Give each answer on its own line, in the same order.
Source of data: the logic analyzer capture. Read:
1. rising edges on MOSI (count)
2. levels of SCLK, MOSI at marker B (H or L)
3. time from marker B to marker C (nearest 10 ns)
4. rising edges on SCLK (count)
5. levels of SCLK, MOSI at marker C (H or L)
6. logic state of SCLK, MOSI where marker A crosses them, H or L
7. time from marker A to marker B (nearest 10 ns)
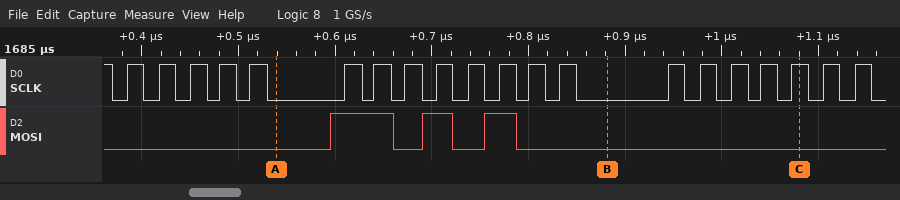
3
SCLK=L, MOSI=L
200 ns
20
SCLK=H, MOSI=L
SCLK=L, MOSI=L
340 ns
